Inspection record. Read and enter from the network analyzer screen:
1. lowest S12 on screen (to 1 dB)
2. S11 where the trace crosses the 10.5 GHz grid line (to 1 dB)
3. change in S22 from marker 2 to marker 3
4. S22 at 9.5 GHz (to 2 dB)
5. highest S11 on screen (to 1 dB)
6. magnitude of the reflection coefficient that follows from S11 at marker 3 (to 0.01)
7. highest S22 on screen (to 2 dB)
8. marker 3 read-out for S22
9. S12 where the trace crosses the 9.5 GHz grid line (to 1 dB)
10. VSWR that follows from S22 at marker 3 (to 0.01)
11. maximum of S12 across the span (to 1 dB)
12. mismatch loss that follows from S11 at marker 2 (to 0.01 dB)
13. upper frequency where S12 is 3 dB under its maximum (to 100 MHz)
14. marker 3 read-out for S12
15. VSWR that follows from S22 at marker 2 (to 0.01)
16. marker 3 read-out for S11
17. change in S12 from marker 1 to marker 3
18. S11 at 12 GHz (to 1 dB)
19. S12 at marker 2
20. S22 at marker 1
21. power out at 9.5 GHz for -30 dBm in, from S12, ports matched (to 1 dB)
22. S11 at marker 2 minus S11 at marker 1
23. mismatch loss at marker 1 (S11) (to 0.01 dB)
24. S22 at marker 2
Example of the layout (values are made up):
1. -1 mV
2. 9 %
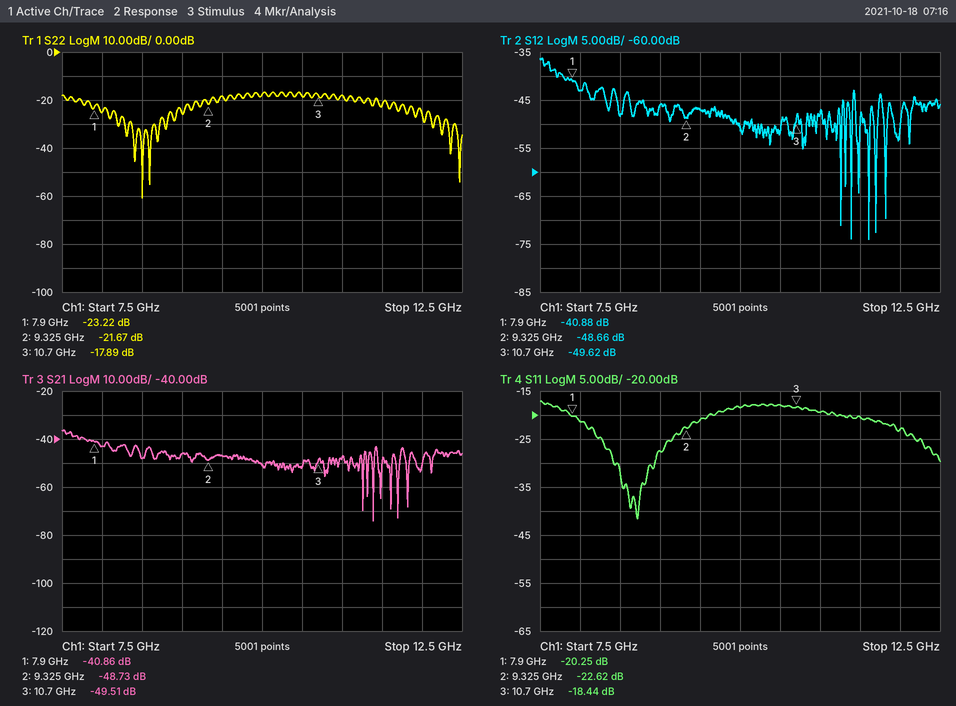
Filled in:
1. -74 dB
2. -18 dB
3. 3.78 dB
4. -18 dB
5. -17 dB
6. 0.12
7. -16 dB
8. -17.89 dB
9. -47 dB
10. 1.29
11. -36 dB
12. 0.02 dB
13. 7.7 GHz
14. -49.62 dB
15. 1.18
16. -18.44 dB
17. -8.74 dB
18. -23 dB
19. -48.66 dB
20. -23.22 dB
21. -77 dBm
22. -2.37 dB
23. 0.04 dB
24. -21.67 dB
